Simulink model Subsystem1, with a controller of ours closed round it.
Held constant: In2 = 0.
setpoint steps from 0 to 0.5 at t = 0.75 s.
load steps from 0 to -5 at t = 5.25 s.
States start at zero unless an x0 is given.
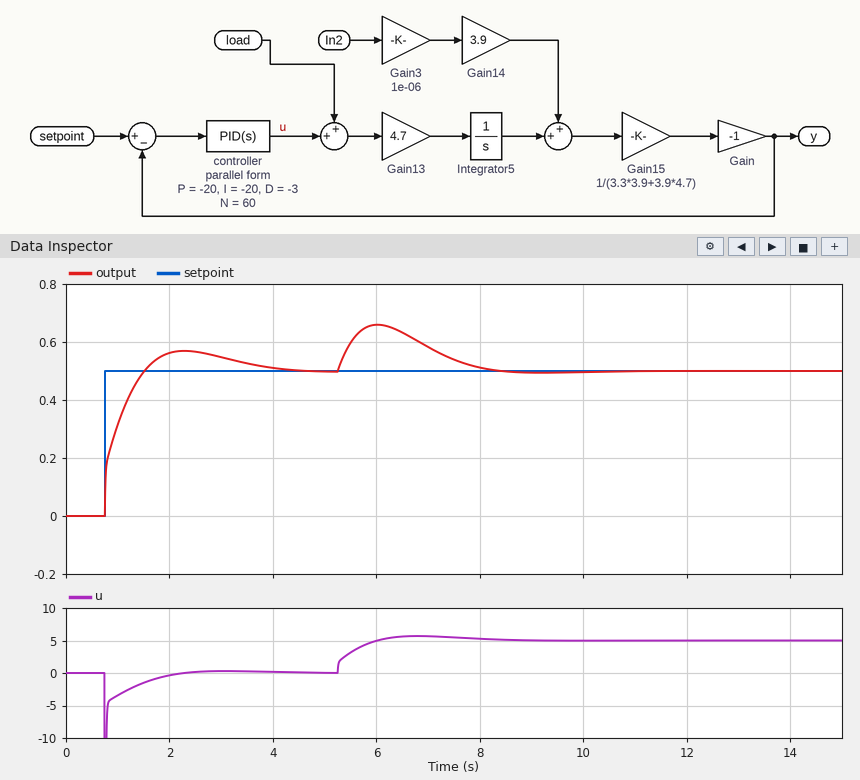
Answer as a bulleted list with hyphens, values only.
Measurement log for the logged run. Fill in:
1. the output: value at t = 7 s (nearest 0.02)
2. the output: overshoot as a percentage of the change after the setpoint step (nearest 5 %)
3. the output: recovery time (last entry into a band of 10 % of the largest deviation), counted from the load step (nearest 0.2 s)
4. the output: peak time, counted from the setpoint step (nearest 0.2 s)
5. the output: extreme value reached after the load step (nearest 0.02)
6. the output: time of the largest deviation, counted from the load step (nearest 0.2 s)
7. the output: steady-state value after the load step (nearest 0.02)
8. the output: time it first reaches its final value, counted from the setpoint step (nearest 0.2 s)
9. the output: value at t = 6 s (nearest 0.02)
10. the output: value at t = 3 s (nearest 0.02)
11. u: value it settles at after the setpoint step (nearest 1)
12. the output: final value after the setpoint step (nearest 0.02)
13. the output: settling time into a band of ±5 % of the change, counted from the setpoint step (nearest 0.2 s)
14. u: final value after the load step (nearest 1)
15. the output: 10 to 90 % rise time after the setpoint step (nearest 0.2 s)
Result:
- 0.58
- 15 %
- 2.6 s
- 1.6 s
- 0.66
- 0.8 s
- 0.50
- 0.8 s
- 0.66
- 0.54
- 0
- 0.50
- 2.8 s
- 5
- 0.6 s
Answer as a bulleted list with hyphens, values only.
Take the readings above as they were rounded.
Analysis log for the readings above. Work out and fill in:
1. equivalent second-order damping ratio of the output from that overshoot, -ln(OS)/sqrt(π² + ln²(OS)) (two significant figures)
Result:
- 0.52
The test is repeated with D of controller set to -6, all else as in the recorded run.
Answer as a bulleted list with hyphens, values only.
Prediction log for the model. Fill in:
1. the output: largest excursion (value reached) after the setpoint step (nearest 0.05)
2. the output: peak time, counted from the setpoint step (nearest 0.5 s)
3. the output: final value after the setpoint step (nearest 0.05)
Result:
- 0.55
- 2.0 s
- 0.50
